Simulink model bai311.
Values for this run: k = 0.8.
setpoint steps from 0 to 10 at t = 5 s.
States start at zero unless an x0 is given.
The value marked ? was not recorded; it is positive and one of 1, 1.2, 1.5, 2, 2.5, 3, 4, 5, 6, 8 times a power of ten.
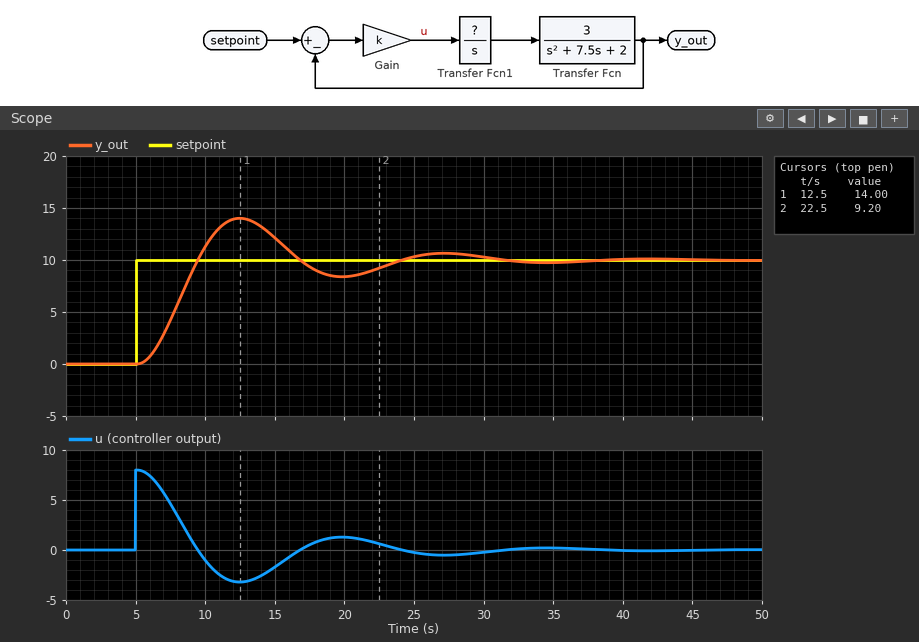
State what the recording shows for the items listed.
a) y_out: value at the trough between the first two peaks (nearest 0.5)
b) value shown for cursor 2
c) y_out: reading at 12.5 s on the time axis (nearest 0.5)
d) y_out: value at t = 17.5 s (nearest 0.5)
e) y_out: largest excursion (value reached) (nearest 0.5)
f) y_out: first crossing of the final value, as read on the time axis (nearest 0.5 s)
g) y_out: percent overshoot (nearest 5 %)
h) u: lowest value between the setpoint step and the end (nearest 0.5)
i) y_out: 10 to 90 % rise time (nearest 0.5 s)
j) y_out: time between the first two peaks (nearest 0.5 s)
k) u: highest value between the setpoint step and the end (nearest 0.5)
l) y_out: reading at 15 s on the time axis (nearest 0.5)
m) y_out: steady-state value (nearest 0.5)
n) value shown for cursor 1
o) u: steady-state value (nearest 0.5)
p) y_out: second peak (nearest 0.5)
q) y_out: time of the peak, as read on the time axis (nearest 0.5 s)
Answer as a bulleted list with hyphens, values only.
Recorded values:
- 8.5
- 9.20
- 14.0
- 9.5
- 14.0
- 9.5 s
- 40 %
- -3.0
- 3.0 s
- 14.5 s
- 8.0
- 12.0
- 10.0
- 14.00
- 0.0
- 10.5
- 12.5 s
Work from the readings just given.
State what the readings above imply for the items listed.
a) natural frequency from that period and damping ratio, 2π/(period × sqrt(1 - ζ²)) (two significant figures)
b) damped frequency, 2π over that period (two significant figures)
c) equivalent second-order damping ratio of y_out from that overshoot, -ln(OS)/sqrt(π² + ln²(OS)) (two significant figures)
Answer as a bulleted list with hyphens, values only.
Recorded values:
- 0.45 rad/s
- 0.43 rad/s
- 0.28
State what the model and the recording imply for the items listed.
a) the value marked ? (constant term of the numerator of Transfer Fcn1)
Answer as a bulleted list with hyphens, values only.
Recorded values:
- 0.6
